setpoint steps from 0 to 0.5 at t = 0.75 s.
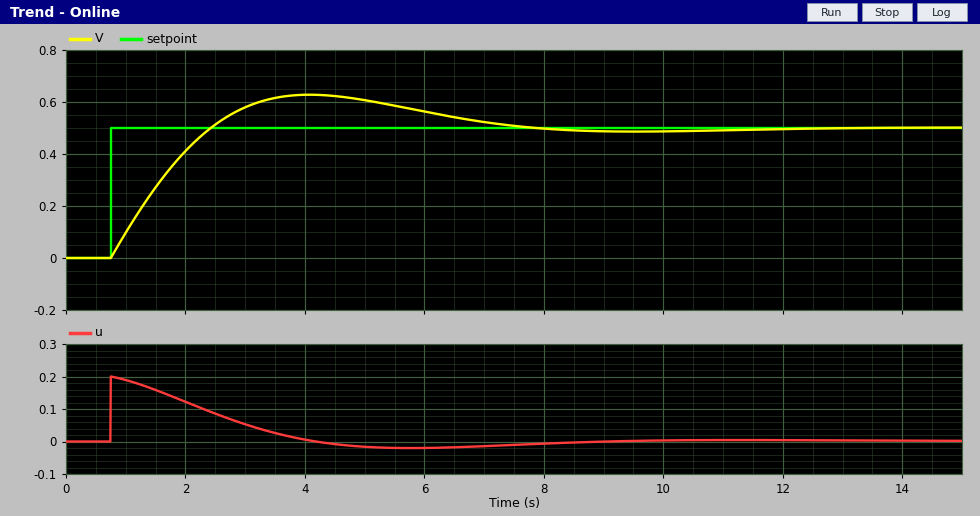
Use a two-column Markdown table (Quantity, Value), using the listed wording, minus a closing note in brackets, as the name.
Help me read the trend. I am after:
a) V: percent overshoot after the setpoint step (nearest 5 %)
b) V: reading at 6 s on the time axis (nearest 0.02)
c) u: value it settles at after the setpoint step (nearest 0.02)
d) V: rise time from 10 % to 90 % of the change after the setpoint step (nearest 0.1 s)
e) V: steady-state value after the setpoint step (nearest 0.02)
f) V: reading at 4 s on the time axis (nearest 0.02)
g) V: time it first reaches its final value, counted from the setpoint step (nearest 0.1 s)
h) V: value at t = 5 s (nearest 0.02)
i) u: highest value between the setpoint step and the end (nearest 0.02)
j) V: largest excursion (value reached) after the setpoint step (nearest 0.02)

| Quantity | Value |
|---|---|
| V: percent overshoot after the setpoint step | 25 % |
| V: reading at 6 s on the time axis | 0.56 |
| u: value it settles at after the setpoint step | 0.00 |
| V: rise time from 10 % to 90 % of the change after the setpoint step | 1.3 s |
| V: steady-state value after the setpoint step | 0.50 |
| V: reading at 4 s on the time axis | 0.62 |
| V: time it first reaches its final value, counted from the setpoint step | 1.7 s |
| V: value at t = 5 s | 0.60 |
| u: highest value between the setpoint step and the end | 0.20 |
| V: largest excursion (value reached) after the setpoint step | 0.62 |
